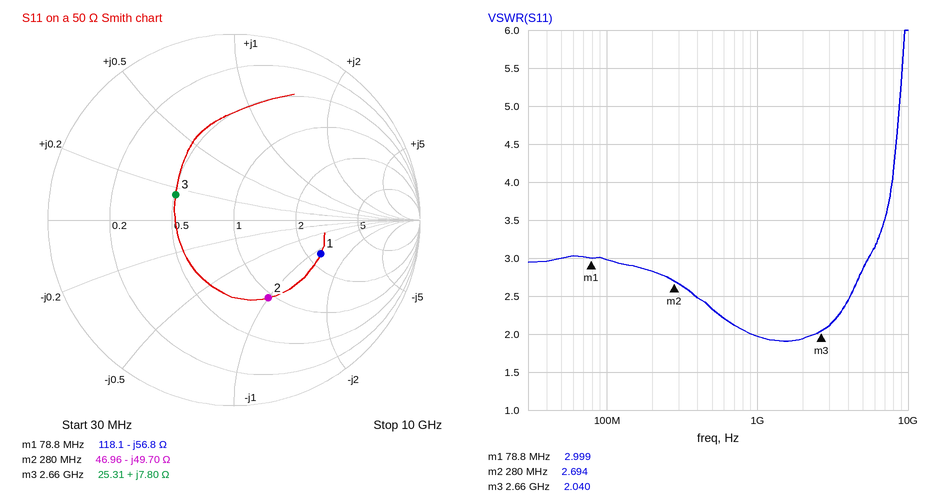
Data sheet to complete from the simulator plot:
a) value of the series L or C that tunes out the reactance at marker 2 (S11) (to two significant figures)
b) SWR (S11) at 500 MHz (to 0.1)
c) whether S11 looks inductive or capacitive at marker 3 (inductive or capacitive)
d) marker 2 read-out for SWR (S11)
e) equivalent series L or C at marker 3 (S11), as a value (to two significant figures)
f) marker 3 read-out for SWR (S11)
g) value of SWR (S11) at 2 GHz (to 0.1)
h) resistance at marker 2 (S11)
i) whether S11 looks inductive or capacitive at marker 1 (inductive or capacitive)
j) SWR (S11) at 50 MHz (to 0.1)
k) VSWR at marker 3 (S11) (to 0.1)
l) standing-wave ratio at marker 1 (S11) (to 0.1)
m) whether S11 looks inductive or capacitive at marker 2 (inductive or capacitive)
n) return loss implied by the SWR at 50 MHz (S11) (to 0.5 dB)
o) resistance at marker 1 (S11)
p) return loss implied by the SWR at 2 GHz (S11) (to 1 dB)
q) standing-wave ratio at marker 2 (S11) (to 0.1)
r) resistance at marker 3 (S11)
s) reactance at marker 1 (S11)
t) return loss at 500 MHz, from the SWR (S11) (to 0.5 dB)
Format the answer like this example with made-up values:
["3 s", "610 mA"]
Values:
["28 nH", "2.3", "inductive", "2.694", "470 pH", "2.040", "1.9", "46.96 Ω", "capacitive", "3.0", "2.0", "3.0", "capacitive", "6.0 dB", "118.1 Ω", "10 dB", "2.7", "25.31 Ω", "-56.8 Ω", "8.0 dB"]
